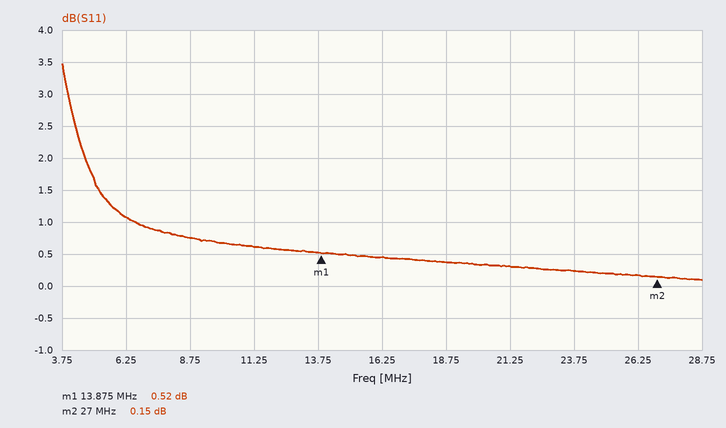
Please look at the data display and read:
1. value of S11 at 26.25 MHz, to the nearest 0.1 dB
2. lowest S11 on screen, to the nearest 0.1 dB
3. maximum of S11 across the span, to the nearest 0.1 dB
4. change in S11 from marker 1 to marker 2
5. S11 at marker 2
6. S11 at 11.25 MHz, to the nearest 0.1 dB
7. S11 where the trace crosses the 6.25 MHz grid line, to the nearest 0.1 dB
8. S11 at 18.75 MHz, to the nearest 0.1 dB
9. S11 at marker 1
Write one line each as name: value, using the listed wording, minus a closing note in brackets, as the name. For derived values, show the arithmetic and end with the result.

value of S11 at 26.25 MHz, to the nearest 0.1 dB: 0.2 dB
lowest S11 on screen, to the nearest 0.1 dB: 0.1 dB
maximum of S11 across the span, to the nearest 0.1 dB: 3.5 dB
change in S11 from marker 1 to marker 2: 0.15 − (0.52) = -0.37 dB
S11 at marker 2: 0.15 dB
S11 at 11.25 MHz, to the nearest 0.1 dB: 0.6 dB
S11 where the trace crosses the 6.25 MHz grid line, to the nearest 0.1 dB: 1.1 dB
S11 at 18.75 MHz, to the nearest 0.1 dB: 0.4 dB
S11 at marker 1: 0.52 dB
